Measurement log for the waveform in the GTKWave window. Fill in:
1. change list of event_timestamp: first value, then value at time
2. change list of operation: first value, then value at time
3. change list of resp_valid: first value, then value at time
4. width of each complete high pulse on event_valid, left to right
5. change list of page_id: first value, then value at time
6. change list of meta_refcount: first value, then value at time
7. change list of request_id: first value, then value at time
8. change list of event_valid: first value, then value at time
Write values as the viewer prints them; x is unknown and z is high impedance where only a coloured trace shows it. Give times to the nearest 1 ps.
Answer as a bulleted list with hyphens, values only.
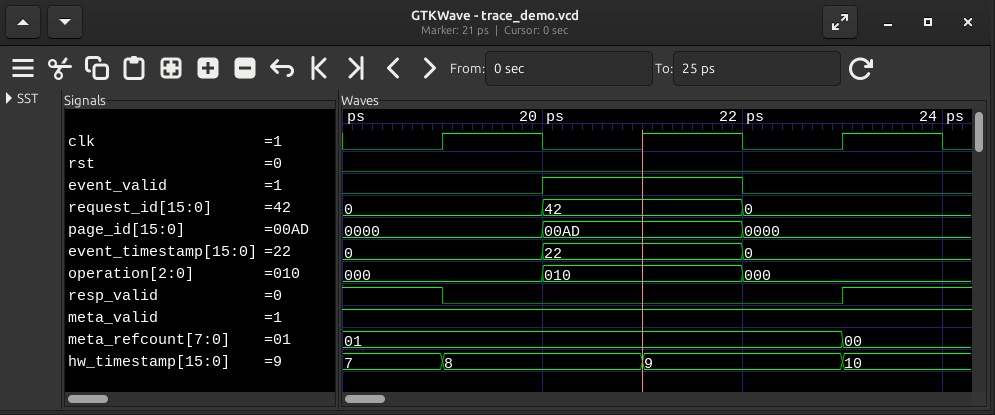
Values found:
- 0, 22 at 20 ps, 0 at 22 ps
- 000, 010 at 20 ps, 000 at 22 ps
- 1, 0 at 19 ps, 1 at 23 ps
- 2 ps
- 0000, 00AD at 20 ps, 0000 at 22 ps
- 01, 00 at 23 ps
- 0, 42 at 20 ps, 0 at 22 ps
- 0, 1 at 20 ps, 0 at 22 ps
